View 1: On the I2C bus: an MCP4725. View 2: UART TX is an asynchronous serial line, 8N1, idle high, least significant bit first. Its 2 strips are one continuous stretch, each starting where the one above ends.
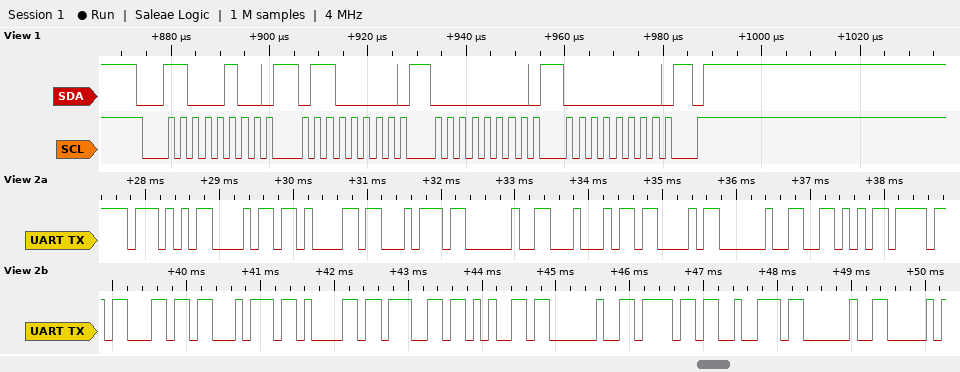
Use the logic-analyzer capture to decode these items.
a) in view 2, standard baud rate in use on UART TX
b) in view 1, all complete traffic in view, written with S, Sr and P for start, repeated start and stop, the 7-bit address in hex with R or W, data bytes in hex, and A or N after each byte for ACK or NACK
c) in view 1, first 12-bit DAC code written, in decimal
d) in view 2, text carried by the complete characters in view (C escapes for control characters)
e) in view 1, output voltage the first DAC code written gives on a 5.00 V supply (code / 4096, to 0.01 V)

9600 baud
S 62W A 60 A 00 A 00 A P
0
"What DC Voltage or "
0.00 V
